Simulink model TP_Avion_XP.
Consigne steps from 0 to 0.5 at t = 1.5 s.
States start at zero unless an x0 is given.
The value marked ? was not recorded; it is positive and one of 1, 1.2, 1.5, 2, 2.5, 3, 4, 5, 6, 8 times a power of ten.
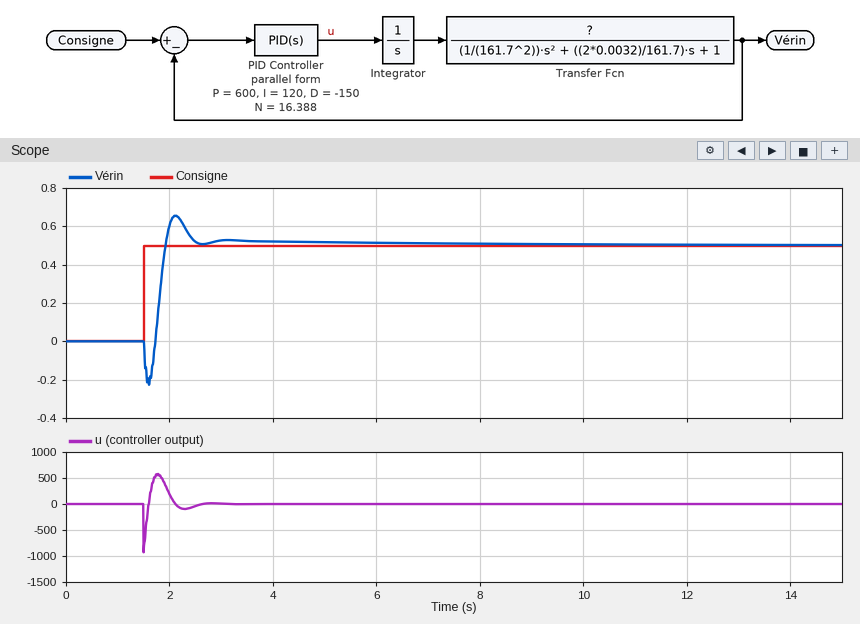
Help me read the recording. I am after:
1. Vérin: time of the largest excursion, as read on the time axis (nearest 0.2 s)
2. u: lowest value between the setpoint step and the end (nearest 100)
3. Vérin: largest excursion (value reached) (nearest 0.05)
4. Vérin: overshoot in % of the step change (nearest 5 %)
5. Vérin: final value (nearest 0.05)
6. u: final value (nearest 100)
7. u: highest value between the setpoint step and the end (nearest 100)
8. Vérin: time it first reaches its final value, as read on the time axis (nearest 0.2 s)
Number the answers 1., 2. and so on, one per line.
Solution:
1. 2.2 s
2. -900
3. 0.65
4. 30 %
5. 0.50
6. 0
7. 600
8. 2.0 s
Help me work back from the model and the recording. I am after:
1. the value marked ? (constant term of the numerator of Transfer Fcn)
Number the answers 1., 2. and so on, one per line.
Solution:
1. 0.005
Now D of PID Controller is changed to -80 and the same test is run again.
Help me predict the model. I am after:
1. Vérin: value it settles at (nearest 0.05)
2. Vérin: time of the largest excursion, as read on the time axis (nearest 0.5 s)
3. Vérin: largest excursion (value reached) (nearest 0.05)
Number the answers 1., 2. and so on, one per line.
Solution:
1. 0.50
2. 2.5 s
3. 0.55
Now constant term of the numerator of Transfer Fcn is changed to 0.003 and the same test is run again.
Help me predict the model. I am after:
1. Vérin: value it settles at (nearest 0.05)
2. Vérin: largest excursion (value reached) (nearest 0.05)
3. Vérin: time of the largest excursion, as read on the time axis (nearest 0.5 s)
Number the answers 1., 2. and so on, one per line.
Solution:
1. 0.50
2. 0.55
3. 3.0 s
